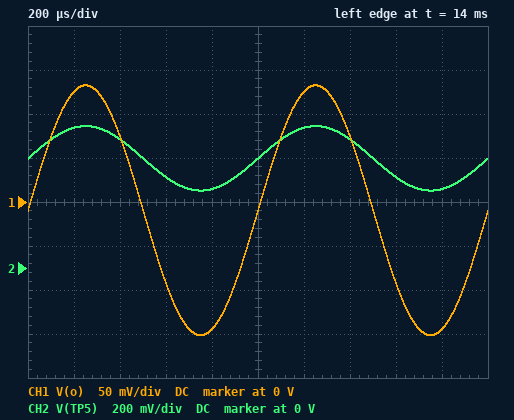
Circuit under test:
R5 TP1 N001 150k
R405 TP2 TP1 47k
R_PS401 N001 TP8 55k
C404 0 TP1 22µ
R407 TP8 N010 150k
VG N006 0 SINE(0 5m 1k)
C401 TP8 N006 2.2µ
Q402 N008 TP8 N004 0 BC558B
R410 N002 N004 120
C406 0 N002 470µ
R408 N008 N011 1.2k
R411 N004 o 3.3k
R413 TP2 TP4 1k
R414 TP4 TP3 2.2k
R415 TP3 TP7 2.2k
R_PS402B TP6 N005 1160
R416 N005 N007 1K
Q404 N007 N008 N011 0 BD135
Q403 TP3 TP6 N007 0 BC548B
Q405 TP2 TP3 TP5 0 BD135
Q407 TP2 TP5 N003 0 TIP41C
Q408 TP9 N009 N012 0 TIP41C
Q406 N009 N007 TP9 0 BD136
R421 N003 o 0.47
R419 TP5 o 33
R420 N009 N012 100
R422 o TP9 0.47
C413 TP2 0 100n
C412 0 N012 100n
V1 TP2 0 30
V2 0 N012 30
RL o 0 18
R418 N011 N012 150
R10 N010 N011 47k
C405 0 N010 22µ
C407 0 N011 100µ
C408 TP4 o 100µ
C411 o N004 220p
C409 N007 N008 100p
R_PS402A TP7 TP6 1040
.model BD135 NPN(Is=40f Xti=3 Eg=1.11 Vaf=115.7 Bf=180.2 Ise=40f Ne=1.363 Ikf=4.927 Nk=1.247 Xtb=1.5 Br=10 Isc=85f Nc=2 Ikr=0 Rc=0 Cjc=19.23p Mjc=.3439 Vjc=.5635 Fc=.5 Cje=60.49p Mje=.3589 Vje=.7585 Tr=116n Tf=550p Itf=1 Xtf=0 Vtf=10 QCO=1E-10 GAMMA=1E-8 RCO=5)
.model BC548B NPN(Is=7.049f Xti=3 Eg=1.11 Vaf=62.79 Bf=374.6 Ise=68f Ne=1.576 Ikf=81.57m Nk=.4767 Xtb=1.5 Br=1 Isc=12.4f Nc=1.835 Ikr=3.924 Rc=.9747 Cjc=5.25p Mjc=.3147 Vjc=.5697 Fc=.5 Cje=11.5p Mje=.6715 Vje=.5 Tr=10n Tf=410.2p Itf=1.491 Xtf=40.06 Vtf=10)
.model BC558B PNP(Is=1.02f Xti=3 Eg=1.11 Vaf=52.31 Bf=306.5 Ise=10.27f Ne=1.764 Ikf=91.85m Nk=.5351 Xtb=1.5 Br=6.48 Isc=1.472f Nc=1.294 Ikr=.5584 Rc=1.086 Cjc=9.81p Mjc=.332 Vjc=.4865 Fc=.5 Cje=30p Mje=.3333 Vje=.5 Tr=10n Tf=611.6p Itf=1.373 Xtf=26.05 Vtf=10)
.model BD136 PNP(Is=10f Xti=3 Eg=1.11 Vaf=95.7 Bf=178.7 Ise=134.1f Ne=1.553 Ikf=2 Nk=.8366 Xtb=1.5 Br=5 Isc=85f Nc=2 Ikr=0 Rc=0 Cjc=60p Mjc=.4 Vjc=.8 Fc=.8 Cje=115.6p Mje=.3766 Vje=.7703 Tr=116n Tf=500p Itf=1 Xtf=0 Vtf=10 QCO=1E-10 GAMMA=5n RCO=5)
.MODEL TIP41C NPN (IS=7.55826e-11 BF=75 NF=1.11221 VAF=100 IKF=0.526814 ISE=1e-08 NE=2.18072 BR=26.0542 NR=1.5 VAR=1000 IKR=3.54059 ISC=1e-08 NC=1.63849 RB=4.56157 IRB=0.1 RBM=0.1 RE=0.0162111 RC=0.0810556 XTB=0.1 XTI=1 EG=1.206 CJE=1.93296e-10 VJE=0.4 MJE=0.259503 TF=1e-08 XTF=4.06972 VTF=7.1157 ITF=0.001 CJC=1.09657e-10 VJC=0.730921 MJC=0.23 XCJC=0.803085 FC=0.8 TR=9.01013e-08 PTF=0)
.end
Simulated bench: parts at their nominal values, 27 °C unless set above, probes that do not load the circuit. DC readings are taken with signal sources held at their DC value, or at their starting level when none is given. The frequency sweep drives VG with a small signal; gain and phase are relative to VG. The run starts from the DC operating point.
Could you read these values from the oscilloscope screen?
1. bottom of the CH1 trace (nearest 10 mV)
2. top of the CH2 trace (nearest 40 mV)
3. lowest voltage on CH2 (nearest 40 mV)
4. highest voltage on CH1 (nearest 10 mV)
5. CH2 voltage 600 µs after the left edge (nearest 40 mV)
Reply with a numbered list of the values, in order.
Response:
1. -150 mV
2. 640 mV
3. 360 mV
4. 130 mV
5. 400 mV
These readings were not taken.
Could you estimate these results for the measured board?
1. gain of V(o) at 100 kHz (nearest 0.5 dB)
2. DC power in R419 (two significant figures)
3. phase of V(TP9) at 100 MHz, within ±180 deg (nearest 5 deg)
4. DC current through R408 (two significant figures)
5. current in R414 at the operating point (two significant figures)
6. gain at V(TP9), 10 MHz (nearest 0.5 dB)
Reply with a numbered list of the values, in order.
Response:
1. 27.0 dB
2. 7.8 mW
3. 75 deg
4. 560 µA
5. 9.0 mA
6. -3.0 dB
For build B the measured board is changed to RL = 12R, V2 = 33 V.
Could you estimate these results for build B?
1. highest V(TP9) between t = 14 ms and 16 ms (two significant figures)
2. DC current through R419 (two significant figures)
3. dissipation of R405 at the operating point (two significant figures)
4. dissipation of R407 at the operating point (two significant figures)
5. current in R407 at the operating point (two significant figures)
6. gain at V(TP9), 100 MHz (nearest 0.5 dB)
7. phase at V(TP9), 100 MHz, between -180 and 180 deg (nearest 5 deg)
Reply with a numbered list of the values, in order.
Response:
1. -1.6 V
2. 14 mA
3. 870 µW
4. 2.8 mW
5. 140 µA
6. -20.5 dB
7. 100 deg
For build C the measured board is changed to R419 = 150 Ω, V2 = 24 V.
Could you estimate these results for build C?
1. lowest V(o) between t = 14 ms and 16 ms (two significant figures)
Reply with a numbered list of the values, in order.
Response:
1. 3.1 V
